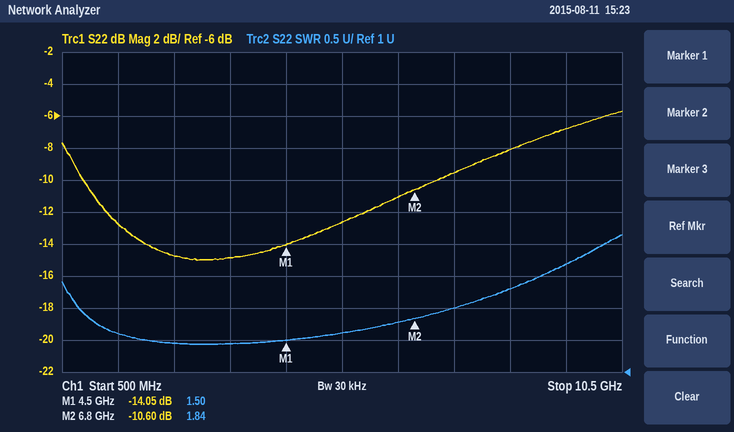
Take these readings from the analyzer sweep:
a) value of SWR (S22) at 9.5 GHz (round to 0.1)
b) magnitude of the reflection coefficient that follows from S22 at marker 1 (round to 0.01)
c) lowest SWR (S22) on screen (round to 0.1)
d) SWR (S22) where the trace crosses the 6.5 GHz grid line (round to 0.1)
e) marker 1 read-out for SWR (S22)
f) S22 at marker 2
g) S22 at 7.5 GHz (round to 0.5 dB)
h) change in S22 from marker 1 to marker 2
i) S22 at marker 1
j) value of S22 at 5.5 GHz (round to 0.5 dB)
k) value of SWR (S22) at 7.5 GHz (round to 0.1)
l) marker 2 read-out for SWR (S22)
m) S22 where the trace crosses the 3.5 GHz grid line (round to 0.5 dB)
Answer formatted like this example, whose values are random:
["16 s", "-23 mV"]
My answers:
["2.7", "0.20", "1.4", "1.8", "1.50", "-10.60 dB", "-9.5 dB", "3.45 dB", "-14.05 dB", "-12.5 dB", "2.0", "1.84", "-15.0 dB"]
